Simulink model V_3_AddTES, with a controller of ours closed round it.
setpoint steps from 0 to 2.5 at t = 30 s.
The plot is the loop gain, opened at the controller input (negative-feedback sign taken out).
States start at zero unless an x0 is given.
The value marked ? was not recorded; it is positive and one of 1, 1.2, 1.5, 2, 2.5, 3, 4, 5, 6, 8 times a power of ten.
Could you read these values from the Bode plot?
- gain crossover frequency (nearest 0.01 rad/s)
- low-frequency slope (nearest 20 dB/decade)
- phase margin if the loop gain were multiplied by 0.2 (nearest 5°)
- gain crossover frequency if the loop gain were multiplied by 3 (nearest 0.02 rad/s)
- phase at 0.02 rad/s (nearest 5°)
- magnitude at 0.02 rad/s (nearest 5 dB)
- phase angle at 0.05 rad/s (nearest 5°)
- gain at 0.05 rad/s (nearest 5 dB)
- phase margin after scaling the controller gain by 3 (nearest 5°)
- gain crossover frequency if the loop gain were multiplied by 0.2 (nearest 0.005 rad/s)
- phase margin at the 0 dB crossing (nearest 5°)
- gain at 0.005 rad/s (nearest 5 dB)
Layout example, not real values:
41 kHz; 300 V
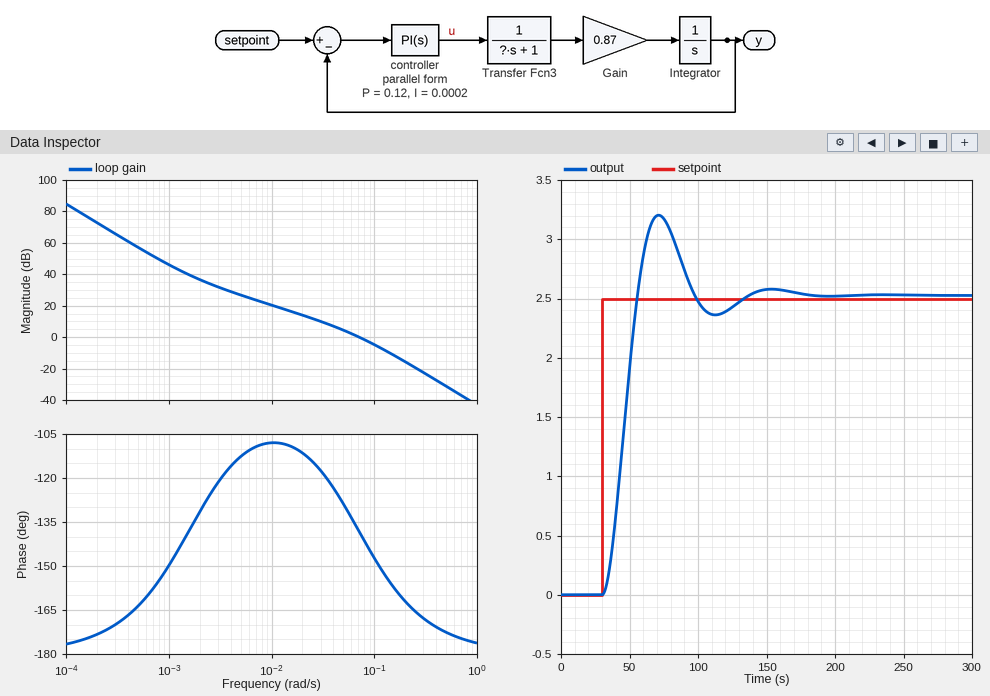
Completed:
0.07 rad/s; -40 dB/decade; 70°; 0.14 rad/s; -110°; 15 dB; -130°; 5 dB; 25°; 0.020 rad/s; 40°; 25 dB
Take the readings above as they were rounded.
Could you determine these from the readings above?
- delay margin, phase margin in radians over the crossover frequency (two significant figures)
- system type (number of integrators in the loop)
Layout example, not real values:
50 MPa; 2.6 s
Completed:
10.0 s; 2
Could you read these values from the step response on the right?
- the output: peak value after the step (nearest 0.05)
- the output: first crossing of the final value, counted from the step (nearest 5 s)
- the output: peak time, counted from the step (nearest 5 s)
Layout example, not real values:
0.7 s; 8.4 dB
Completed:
3.20; 25 s; 40 s
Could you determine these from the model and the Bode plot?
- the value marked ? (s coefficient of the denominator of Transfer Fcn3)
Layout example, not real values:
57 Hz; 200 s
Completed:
15
